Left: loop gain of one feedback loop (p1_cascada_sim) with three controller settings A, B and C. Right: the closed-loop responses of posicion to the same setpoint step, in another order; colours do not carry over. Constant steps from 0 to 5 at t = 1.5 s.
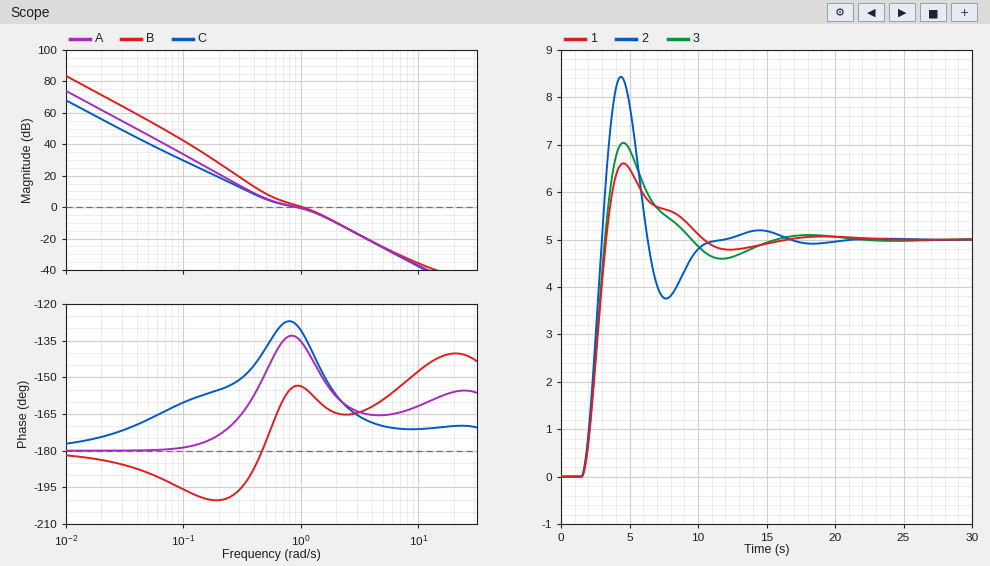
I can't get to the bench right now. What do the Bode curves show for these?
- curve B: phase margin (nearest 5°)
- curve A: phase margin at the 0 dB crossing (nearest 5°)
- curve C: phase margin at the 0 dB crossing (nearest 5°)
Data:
25°
45°
50°
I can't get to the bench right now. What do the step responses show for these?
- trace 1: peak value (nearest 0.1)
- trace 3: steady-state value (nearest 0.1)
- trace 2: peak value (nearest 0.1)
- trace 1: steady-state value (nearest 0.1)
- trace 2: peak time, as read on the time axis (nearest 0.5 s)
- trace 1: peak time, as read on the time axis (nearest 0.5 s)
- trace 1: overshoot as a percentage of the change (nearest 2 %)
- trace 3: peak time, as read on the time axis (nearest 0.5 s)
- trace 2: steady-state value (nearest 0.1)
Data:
6.6
5.0
8.4
5.0
4.5 s
4.5 s
32 %
4.5 s
5.0
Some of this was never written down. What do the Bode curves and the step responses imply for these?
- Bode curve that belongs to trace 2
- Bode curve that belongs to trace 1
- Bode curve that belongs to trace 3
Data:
B
C
A
